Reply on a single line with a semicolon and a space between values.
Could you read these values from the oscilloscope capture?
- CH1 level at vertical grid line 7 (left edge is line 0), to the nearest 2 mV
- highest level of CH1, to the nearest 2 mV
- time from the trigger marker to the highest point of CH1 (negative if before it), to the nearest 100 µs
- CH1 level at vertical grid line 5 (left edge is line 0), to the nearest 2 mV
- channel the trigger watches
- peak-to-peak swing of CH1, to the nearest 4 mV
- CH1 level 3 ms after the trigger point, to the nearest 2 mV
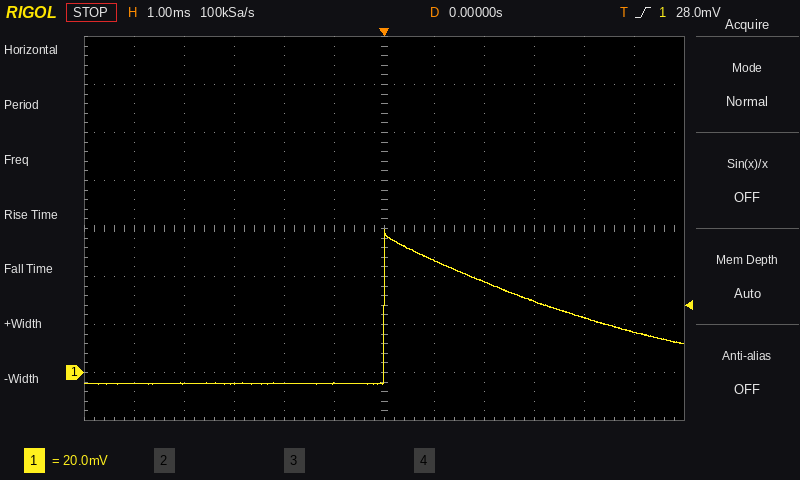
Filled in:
46 mV; 60 mV; 0.0 ms; -4 mV; CH1; 64 mV; 30 mV
